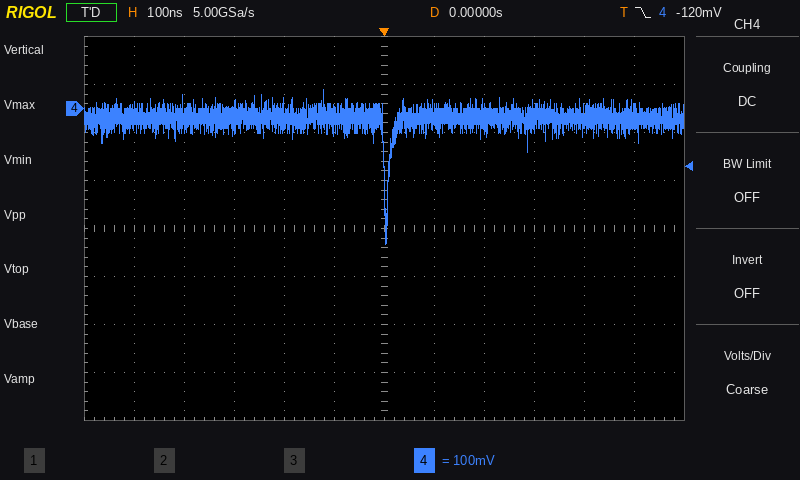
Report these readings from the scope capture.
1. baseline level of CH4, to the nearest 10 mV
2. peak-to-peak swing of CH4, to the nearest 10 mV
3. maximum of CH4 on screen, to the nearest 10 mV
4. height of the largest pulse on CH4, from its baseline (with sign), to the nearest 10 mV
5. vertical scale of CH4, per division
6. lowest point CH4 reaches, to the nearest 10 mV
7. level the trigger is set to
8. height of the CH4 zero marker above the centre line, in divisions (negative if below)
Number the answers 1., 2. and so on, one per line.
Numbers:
1. -20 mV
2. 320 mV
3. 40 mV
4. -260 mV
5. 100 mV
6. -280 mV
7. -120 mV
8. +2.5 div
